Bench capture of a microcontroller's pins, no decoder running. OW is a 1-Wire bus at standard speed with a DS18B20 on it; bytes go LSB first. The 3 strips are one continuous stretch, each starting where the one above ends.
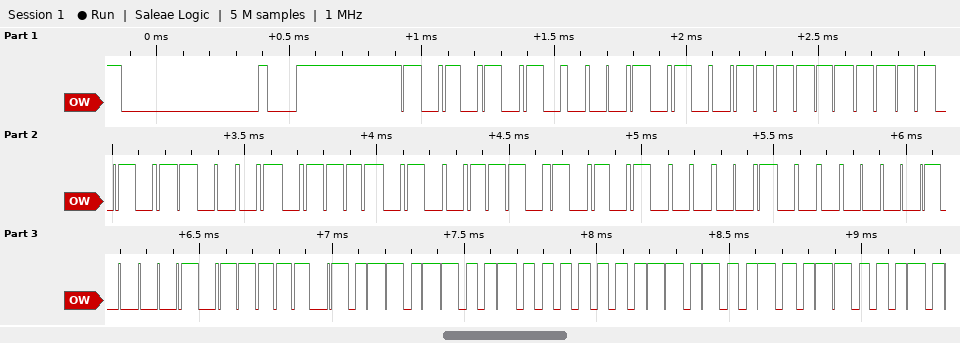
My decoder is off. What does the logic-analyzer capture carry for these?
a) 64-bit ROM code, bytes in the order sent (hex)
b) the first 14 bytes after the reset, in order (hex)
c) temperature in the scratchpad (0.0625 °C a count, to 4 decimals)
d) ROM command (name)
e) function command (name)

28 FF 6B F4 72 15 04 84
55 28 FF 6B F4 72 15 04 84 BE 36 01 4B 46
19.3750 °C
Match ROM
Read Scratchpad
